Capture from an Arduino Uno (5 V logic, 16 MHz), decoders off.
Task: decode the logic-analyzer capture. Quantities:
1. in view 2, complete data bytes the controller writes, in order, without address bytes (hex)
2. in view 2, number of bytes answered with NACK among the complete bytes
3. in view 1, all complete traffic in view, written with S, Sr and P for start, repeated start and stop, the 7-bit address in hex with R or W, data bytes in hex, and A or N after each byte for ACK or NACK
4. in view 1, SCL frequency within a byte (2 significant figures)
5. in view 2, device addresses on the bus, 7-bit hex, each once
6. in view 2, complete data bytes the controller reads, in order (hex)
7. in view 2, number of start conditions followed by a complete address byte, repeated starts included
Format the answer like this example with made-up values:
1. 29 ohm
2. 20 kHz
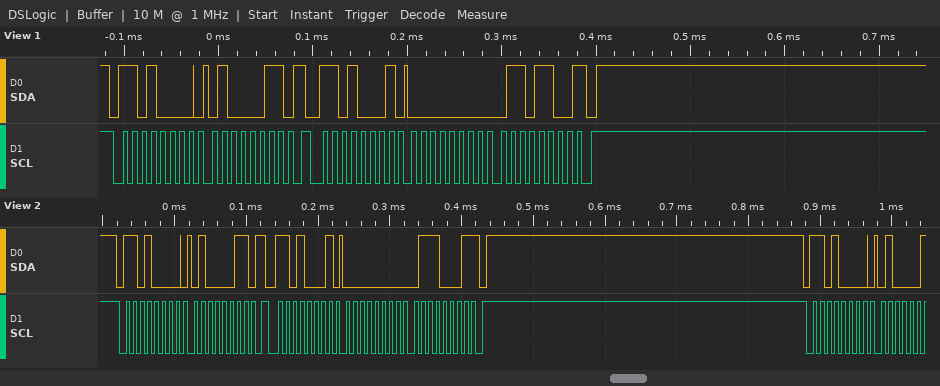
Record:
1. 43
2. 1
3. S 68W A 43 A Sr 68R A 00 A 6C N P
4. 100 kHz
5. 0x68
6. 00 71
7. 3
